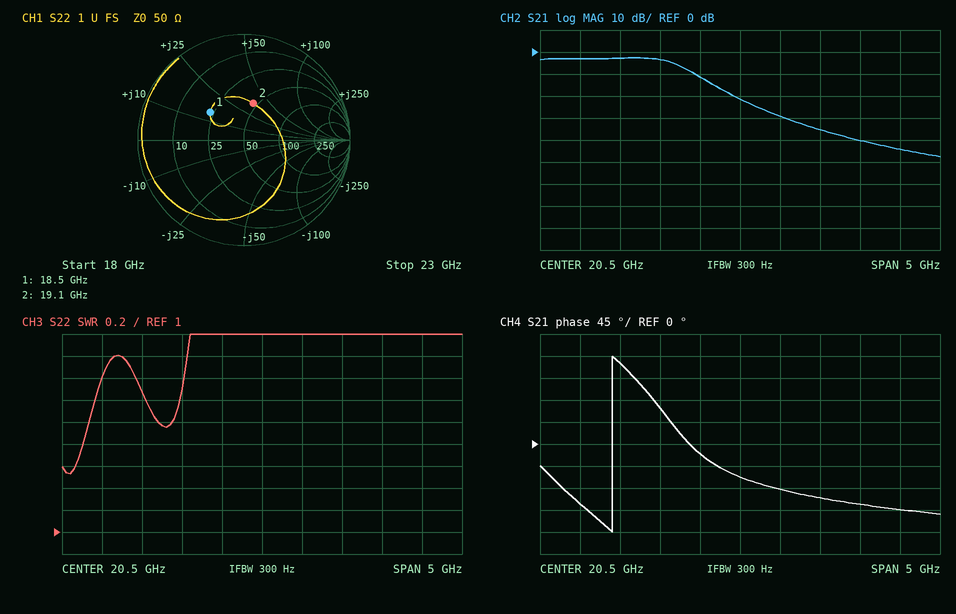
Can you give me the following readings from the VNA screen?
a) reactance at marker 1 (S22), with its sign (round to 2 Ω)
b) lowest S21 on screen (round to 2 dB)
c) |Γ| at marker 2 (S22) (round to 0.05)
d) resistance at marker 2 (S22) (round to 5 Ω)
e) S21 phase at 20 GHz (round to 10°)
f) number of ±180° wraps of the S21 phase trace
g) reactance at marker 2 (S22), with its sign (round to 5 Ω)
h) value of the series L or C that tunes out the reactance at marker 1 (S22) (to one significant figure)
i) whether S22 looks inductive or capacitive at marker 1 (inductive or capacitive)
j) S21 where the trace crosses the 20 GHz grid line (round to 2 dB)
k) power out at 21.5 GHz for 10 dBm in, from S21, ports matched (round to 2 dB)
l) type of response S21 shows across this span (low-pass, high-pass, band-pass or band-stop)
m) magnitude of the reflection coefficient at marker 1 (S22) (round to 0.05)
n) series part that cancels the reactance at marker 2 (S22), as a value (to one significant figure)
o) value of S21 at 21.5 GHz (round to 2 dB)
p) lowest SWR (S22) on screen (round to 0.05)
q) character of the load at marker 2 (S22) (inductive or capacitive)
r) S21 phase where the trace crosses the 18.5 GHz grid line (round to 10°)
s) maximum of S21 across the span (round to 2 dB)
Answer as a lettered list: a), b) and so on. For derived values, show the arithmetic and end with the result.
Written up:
a) +14 Ω
b) -48 dB
c) 0.35
d) 45 Ω
e) -20°
f) 1
g) +35 Ω
h) C = 1/(2π × 18.5 GHz × 14 Ω) ≈ 614 fF, so 600 fF to one significant figure
i) inductive
j) -12 dB
k) 10 dBm + (-36 dB) = -26 dBm
l) low-pass
m) 0.40
n) C = 1/(2π × 19.1 GHz × 35 Ω) ≈ 238 fF, so 200 fF to one significant figure
o) -36 dB
p) 1.55
q) inductive
r) -120°
s) -2 dB
